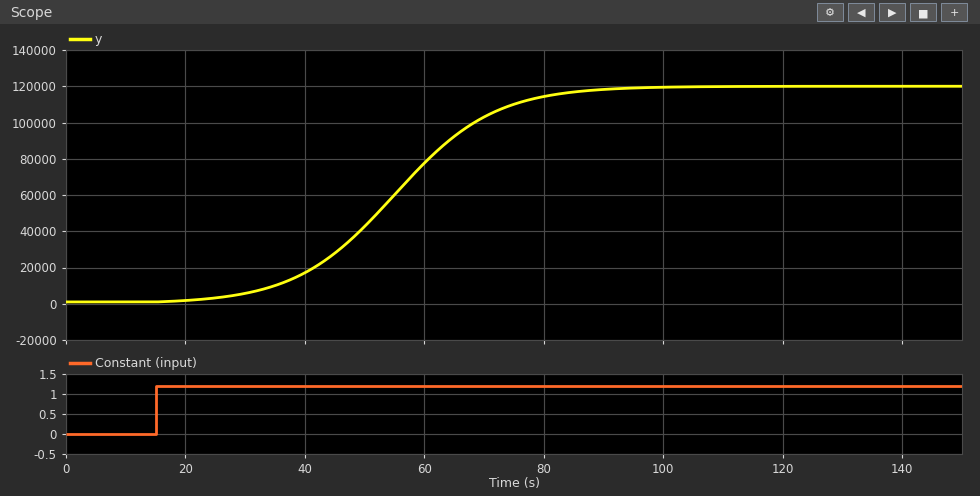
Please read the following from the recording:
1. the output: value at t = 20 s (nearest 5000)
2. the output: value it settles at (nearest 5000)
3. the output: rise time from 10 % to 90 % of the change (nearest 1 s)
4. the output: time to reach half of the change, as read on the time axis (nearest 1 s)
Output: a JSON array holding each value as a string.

["0", "120000", "36 s", "55 s"]
